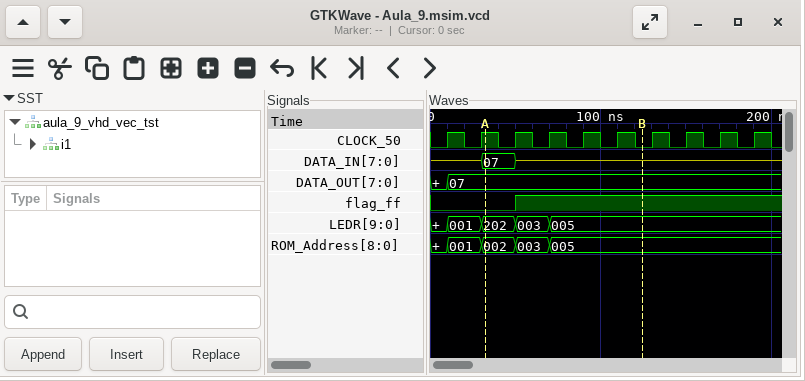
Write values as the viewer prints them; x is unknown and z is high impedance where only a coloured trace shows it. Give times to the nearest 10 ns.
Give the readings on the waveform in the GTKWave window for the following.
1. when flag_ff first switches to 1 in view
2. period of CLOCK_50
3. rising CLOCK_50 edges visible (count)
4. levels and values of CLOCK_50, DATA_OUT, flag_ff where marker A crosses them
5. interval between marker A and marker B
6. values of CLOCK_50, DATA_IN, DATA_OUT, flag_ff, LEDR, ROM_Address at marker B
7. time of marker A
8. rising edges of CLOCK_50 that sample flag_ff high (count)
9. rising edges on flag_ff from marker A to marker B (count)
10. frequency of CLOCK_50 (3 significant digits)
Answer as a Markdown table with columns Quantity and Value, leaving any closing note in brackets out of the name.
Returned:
| Quantity | Value |
|---|---|
| when flag_ff first switches to 1 in view | 50 ns |
| period of CLOCK_50 | 20 ns |
| rising CLOCK_50 edges visible | 10 |
| levels and values of CLOCK_50, DATA_OUT, flag_ff where marker A crosses them | CLOCK_50=1, DATA_OUT=07, flag_ff=0 |
| interval between marker A and marker B | 90 ns |
| values of CLOCK_50, DATA_IN, DATA_OUT, flag_ff, LEDR, ROM_Address at marker B | CLOCK_50=0, DATA_IN=z, DATA_OUT=07, flag_ff=1, LEDR=005, ROM_Address=005 |
| time of marker A | 30 ns |
| rising edges of CLOCK_50 that sample flag_ff high | 7 |
| rising edges on flag_ff from marker A to marker B | 1 |
| frequency of CLOCK_50 | 50.0 MHz |
